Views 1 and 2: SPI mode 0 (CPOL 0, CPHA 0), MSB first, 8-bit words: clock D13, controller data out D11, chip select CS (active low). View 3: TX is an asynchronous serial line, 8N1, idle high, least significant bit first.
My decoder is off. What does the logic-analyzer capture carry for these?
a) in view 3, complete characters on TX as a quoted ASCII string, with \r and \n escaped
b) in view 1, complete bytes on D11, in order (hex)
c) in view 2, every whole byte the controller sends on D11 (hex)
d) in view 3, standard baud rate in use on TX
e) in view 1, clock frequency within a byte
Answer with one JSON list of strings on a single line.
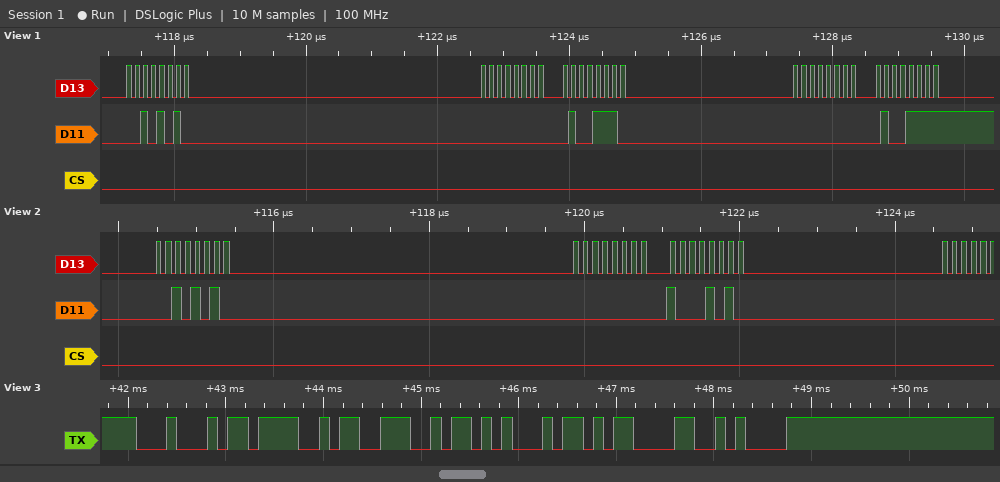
["\"DONE\\r\\n\"", "2A 00 4E 00 4F", "2A 00 8A", "9600 baud", "8 MHz"]
